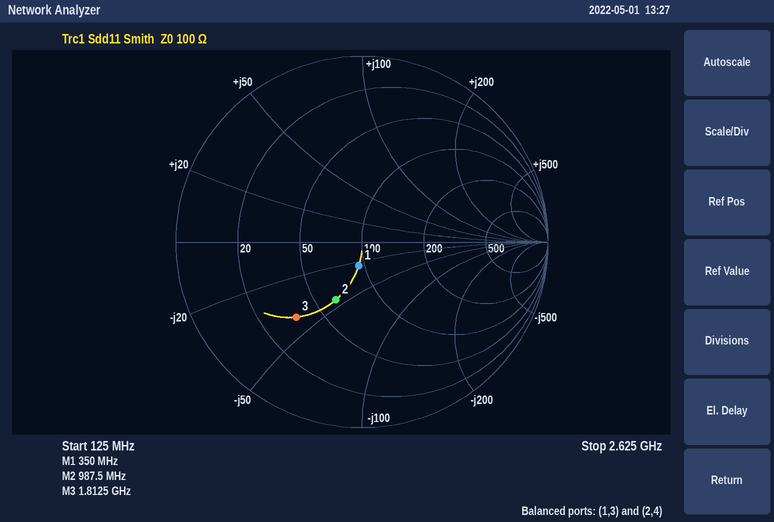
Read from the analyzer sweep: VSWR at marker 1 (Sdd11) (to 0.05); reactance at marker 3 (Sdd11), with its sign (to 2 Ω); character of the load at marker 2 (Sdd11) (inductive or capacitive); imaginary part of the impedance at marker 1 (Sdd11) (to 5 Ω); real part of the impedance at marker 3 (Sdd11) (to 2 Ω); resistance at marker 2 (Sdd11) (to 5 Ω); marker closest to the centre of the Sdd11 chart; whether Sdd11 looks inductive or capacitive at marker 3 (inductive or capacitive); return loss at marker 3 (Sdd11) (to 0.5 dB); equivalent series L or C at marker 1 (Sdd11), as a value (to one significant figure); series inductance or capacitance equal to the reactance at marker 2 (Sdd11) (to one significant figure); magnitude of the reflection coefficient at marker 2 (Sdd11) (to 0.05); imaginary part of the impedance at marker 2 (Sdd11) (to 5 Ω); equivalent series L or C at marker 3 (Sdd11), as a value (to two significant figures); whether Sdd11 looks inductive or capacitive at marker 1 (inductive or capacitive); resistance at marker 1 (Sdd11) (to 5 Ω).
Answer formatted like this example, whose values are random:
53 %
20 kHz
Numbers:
1.30
-40 Ω
capacitive
-25 Ω
36 Ω
65 Ω
marker 1
capacitive
5.5 dB
20 pF
4 pF
0.35
-45 Ω
2.2 pF
capacitive
95 Ω
